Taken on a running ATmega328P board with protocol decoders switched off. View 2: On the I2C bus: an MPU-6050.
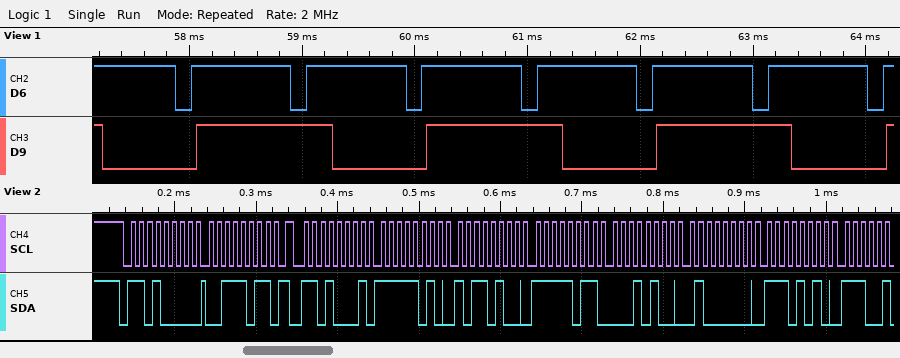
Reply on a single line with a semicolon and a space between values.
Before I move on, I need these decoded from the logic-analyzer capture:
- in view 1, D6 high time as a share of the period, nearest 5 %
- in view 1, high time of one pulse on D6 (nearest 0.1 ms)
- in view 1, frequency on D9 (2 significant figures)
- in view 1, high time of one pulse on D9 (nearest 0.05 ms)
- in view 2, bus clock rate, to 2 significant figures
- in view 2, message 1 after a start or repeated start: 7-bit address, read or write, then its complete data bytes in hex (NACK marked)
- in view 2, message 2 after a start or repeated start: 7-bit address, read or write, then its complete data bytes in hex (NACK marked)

85 %; 0.9 ms; 490 Hz; 1.20 ms; 100 kHz; 0x68 write: 3B; 0x68 read: FA B4 FB 14 40 EA
